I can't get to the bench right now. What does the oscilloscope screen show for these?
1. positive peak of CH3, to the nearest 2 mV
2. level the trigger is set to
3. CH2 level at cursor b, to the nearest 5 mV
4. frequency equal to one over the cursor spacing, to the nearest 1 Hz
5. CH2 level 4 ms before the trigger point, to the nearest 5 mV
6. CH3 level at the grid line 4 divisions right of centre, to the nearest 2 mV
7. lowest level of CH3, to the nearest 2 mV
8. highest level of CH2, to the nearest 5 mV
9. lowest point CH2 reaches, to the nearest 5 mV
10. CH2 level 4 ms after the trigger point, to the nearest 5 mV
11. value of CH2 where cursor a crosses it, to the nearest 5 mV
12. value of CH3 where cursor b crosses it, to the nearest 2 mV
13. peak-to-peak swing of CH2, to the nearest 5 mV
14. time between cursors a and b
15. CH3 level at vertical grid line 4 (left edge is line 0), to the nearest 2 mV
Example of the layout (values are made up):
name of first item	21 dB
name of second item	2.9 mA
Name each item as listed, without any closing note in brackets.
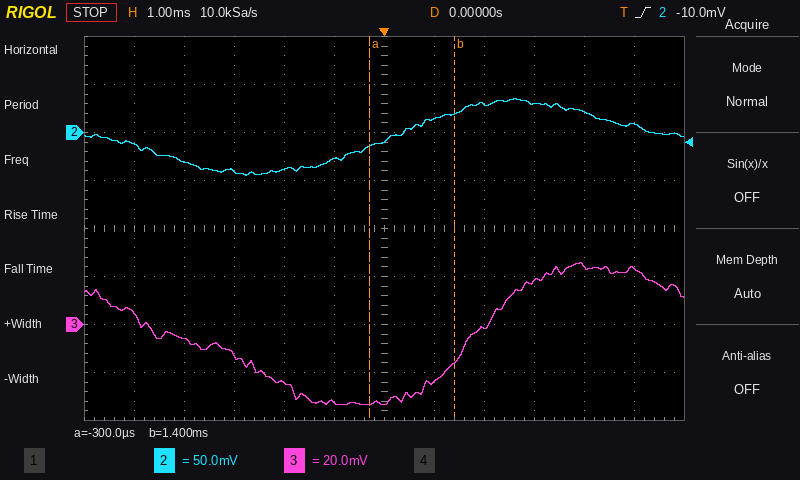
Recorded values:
positive peak of CH3, to the nearest 2 mV	26 mV
level the trigger is set to	-10.0 mV
CH2 level at cursor b, to the nearest 5 mV	20 mV
frequency equal to one over the cursor spacing, to the nearest 1 Hz	588 Hz
CH2 level 4 ms before the trigger point, to the nearest 5 mV	-30 mV
CH3 level at the grid line 4 divisions right of centre, to the nearest 2 mV	24 mV
lowest level of CH3, to the nearest 2 mV	-34 mV
highest level of CH2, to the nearest 5 mV	35 mV
lowest point CH2 reaches, to the nearest 5 mV	-45 mV
CH2 level 4 ms after the trigger point, to the nearest 5 mV	20 mV
value of CH2 where cursor a crosses it, to the nearest 5 mV	-15 mV
value of CH3 where cursor b crosses it, to the nearest 2 mV	-16 mV
peak-to-peak swing of CH2, to the nearest 5 mV	80 mV
time between cursors a and b	1.7 ms
CH3 level at vertical grid line 4 (left edge is line 0), to the nearest 2 mV	-24 mV
